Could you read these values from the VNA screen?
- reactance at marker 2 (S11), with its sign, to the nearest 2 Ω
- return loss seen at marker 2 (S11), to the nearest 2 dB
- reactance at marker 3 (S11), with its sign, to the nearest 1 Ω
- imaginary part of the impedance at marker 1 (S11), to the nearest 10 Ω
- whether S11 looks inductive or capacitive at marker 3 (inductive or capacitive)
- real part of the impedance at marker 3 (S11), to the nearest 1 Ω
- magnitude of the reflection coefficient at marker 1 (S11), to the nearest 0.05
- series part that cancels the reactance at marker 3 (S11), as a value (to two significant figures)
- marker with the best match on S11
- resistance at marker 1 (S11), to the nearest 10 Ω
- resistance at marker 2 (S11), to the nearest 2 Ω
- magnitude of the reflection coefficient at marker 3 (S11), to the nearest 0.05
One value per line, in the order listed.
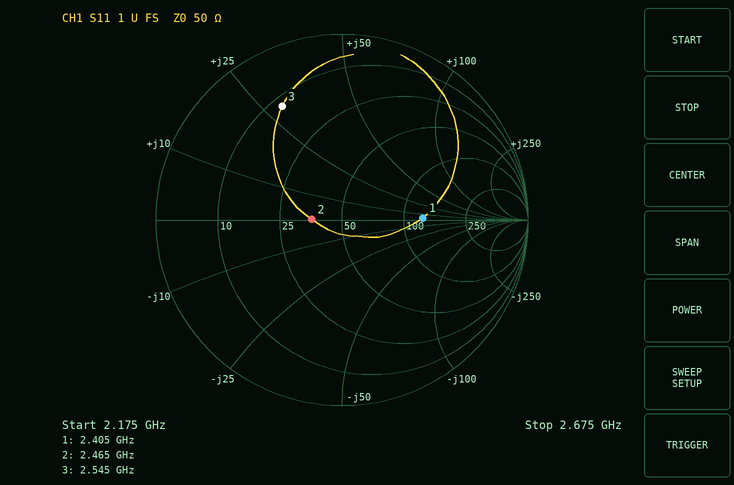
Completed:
0 Ω
16 dB
+29 Ω
0 Ω
inductive
12 Ω
0.45
2.2 pF
marker 2
130 Ω
36 Ω
0.70
